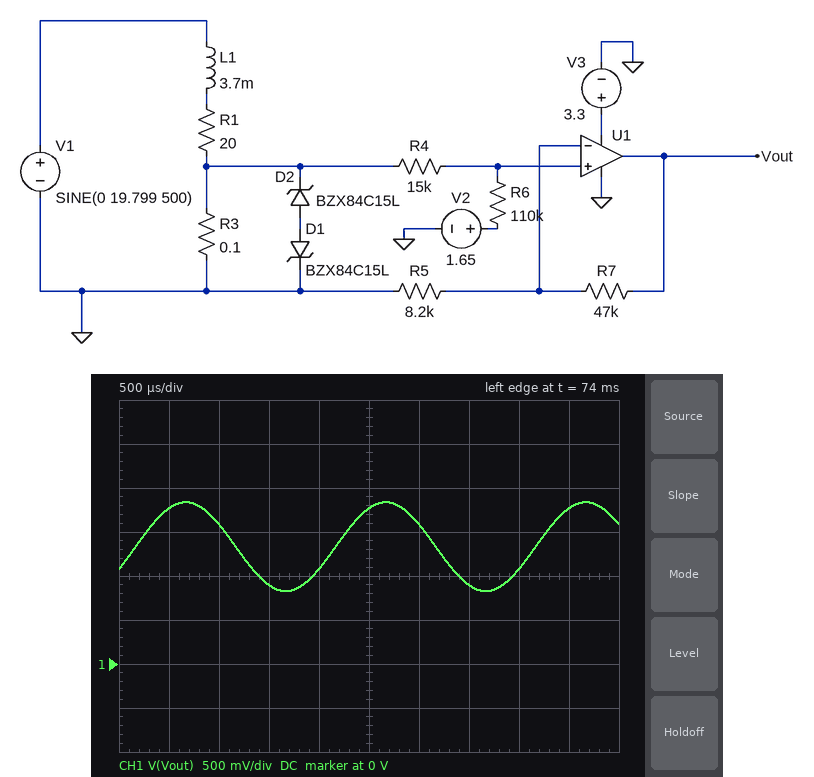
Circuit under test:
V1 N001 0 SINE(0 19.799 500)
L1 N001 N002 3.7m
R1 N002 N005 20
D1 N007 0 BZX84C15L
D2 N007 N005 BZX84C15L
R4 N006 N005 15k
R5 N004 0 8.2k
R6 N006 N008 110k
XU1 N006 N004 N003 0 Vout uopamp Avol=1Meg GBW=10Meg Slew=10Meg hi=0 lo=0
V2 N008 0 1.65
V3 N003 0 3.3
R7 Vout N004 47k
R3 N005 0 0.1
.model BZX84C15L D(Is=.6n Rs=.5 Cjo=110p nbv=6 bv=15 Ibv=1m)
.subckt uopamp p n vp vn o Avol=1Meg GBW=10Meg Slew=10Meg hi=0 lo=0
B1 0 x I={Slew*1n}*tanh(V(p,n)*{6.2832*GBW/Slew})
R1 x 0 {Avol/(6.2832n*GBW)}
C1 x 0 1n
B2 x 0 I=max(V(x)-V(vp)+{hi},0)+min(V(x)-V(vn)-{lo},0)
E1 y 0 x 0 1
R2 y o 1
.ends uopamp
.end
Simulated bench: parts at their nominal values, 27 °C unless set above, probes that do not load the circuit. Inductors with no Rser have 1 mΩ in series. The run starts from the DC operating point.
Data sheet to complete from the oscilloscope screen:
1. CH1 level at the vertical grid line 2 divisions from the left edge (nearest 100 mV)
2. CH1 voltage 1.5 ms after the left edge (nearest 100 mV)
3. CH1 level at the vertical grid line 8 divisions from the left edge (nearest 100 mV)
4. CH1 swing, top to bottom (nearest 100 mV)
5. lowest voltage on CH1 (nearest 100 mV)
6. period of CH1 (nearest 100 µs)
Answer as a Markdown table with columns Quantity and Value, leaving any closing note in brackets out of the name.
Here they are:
| Quantity | Value |
|---|---|
| CH1 level at the vertical grid line 2 divisions from the left edge | 1.6 V |
| CH1 voltage 1.5 ms after the left edge | 900 mV |
| CH1 level at the vertical grid line 8 divisions from the left edge | 1.1 V |
| CH1 swing, top to bottom | 1.0 V |
| lowest voltage on CH1 | 800 mV |
| period of CH1 | 2.0 ms |
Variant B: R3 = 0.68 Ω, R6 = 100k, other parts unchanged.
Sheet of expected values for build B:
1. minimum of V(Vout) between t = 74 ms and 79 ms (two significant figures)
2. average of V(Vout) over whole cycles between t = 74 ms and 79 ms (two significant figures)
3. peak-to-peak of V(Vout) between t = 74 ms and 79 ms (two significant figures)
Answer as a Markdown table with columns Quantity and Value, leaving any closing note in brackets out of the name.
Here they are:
| Quantity | Value |
|---|---|
| minimum of V(Vout) between t = 74 ms and 79 ms | -9.4 mV |
| average of V(Vout) over whole cycles between t = 74 ms and 79 ms | 1.6 V |
| peak-to-peak of V(Vout) between t = 74 ms and 79 ms | 3.3 V |
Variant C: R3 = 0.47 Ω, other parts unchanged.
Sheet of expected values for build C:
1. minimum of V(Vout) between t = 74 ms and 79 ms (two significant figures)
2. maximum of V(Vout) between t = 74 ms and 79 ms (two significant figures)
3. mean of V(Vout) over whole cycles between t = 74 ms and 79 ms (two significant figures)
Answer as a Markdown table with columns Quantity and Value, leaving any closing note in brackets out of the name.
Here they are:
| Quantity | Value |
|---|---|
| minimum of V(Vout) between t = 74 ms and 79 ms | -7.3 mV |
| maximum of V(Vout) between t = 74 ms and 79 ms | 3.3 V |
| mean of V(Vout) over whole cycles between t = 74 ms and 79 ms | 1.5 V |
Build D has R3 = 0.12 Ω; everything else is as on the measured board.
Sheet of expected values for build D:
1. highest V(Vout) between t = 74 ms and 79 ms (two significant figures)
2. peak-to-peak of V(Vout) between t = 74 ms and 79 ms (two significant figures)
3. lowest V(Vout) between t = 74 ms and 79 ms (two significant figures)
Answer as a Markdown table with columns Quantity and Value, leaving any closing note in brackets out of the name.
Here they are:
| Quantity | Value |
|---|---|
| highest V(Vout) between t = 74 ms and 79 ms | 1.9 V |
| peak-to-peak of V(Vout) between t = 74 ms and 79 ms | 1.2 V |
| lowest V(Vout) between t = 74 ms and 79 ms | 730 mV |
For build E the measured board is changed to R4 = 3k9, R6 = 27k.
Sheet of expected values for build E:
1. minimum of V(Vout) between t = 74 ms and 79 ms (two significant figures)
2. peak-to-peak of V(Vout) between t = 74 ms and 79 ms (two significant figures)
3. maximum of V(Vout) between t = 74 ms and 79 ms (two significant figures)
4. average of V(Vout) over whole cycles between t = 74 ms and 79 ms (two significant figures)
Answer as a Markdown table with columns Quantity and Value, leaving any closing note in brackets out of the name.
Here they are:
| Quantity | Value |
|---|---|
| minimum of V(Vout) between t = 74 ms and 79 ms | 900 mV |
| peak-to-peak of V(Vout) between t = 74 ms and 79 ms | 1.0 V |
| maximum of V(Vout) between t = 74 ms and 79 ms | 1.9 V |
| average of V(Vout) over whole cycles between t = 74 ms and 79 ms | 1.4 V |
